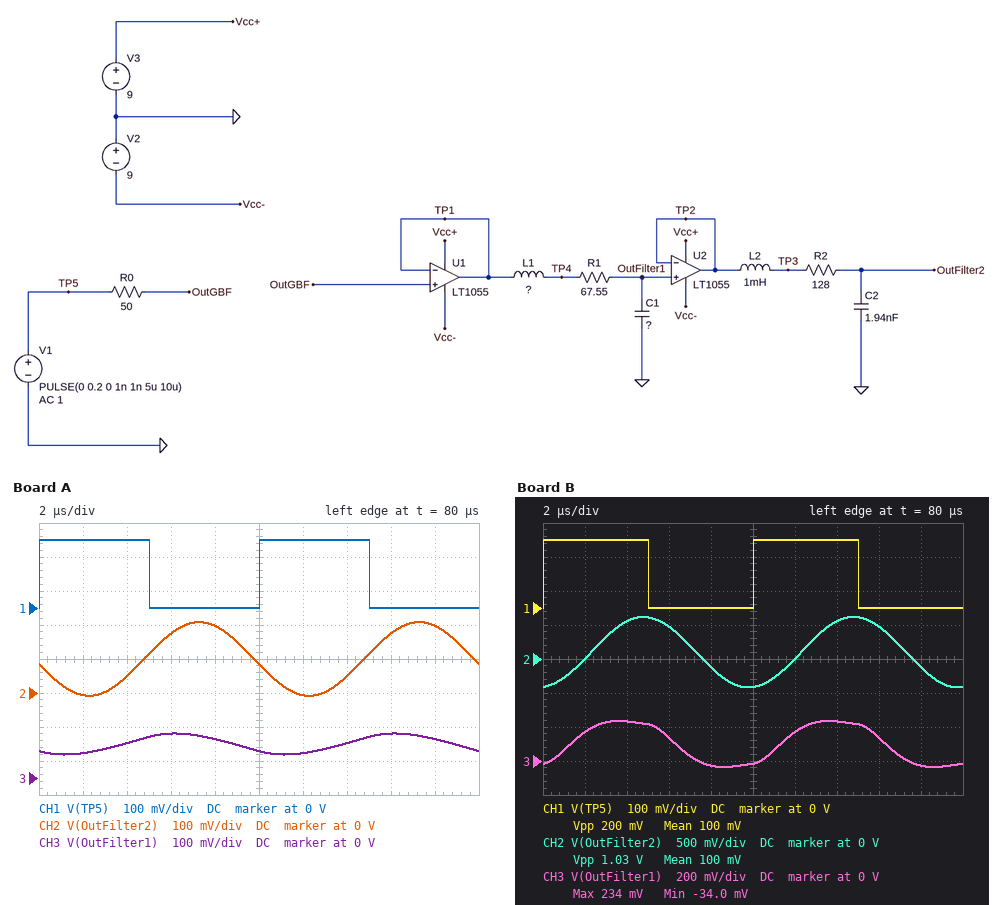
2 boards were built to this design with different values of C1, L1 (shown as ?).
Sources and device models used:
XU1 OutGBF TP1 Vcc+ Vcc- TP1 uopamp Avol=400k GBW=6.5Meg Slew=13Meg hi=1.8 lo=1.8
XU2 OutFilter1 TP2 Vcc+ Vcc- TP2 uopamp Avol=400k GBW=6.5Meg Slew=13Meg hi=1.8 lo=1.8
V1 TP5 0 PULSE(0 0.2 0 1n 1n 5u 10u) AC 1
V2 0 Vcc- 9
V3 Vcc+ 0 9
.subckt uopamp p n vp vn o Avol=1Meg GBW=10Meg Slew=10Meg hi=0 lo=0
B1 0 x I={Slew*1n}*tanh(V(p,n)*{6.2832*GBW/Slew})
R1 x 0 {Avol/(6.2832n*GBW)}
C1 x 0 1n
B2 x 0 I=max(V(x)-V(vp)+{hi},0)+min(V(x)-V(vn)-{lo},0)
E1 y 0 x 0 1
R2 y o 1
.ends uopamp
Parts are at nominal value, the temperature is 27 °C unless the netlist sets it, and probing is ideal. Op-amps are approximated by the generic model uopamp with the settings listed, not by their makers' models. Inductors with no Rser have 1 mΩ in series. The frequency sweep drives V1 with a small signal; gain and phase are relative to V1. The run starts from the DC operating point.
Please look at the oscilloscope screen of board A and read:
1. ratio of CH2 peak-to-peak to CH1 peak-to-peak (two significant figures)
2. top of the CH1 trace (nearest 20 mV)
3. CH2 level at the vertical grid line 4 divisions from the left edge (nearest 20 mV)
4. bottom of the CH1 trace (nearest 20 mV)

1.1
200 mV
200 mV
0 V
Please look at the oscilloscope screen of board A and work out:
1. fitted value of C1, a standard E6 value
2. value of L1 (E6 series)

68 nF
150 µH
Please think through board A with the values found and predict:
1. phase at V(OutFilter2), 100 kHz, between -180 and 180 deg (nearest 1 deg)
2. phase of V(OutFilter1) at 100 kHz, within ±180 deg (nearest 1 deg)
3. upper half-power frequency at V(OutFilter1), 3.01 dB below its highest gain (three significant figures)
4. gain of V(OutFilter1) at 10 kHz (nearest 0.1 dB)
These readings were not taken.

-172 deg
-137 deg
49.0 kHz
0 dB
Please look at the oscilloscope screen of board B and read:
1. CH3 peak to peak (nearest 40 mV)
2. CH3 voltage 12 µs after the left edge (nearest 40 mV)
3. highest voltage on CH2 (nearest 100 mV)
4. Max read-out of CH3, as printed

280 mV
160 mV
600 mV
234 mV
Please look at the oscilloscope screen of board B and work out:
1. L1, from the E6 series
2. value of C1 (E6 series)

68 µH
15 nF
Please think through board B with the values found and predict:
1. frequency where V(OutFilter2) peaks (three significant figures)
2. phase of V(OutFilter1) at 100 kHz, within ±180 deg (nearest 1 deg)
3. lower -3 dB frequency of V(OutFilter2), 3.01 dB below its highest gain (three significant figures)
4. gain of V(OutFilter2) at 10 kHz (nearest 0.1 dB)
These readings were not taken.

113 kHz
-48 deg
103 kHz
0.1 dB
